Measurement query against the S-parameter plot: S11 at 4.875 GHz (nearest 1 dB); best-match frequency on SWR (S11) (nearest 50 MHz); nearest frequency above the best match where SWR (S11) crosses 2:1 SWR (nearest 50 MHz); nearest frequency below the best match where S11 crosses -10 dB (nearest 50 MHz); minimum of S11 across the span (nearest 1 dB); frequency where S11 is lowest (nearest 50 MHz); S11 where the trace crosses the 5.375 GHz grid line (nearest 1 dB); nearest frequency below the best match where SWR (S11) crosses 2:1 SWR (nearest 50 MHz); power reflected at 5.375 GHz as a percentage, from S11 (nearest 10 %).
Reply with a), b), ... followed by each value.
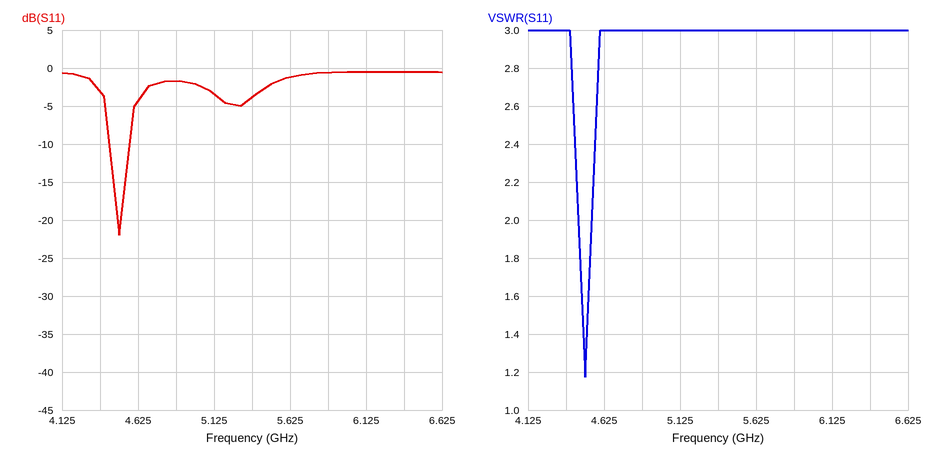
a) -2 dB
b) 4.50 GHz
c) 4.55 GHz
d) 4.45 GHz
e) -22 dB
f) 4.50 GHz
g) -4 dB
h) 4.45 GHz
i) 40 %
